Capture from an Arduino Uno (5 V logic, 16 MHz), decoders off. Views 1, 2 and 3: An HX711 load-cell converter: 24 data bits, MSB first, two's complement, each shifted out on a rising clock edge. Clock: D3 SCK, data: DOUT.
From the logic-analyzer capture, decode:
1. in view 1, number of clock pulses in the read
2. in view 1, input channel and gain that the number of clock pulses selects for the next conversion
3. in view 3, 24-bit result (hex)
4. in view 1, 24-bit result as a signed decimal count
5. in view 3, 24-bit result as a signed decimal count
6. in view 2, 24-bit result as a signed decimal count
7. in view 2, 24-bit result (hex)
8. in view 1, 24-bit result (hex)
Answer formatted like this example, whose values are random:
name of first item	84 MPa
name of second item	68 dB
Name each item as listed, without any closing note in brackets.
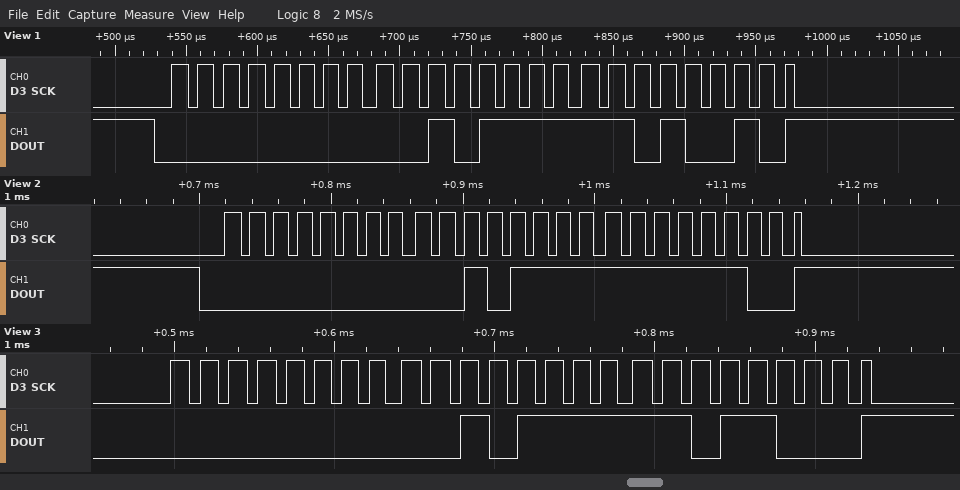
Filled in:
in view 1, number of clock pulses in the read	25
in view 1, input channel and gain that the number of clock pulses selects for the next conversion	channel A, gain 128
in view 3, 24-bit result	0x002FD8
in view 1, 24-bit result as a signed decimal count	12242
in view 3, 24-bit result as a signed decimal count	12248
in view 2, 24-bit result as a signed decimal count	12284
in view 2, 24-bit result	0x002FFC
in view 1, 24-bit result	0x002FD2
